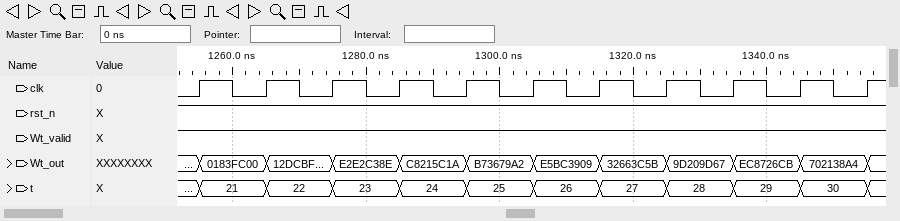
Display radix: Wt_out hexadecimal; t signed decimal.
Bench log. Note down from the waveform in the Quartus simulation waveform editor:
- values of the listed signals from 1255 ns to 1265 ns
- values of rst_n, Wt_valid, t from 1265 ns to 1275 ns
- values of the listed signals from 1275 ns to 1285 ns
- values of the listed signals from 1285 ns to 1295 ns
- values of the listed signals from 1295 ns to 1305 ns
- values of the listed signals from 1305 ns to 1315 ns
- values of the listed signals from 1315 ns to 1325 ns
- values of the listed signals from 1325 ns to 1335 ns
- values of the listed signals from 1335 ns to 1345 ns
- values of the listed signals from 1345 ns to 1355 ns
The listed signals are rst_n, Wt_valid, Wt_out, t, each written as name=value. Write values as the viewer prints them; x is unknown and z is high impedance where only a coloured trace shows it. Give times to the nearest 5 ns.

rst_n=1, Wt_valid=1, Wt_out=0183FC00, t=21
rst_n=1, Wt_valid=1, t=22
rst_n=1, Wt_valid=1, Wt_out=E2E2C38E, t=23
rst_n=1, Wt_valid=1, Wt_out=C8215C1A, t=24
rst_n=1, Wt_valid=1, Wt_out=B73679A2, t=25
rst_n=1, Wt_valid=1, Wt_out=E5BC3909, t=26
rst_n=1, Wt_valid=1, Wt_out=32663C5B, t=27
rst_n=1, Wt_valid=1, Wt_out=9D209D67, t=28
rst_n=1, Wt_valid=1, Wt_out=EC8726CB, t=29
rst_n=1, Wt_valid=1, Wt_out=702138A4, t=30
